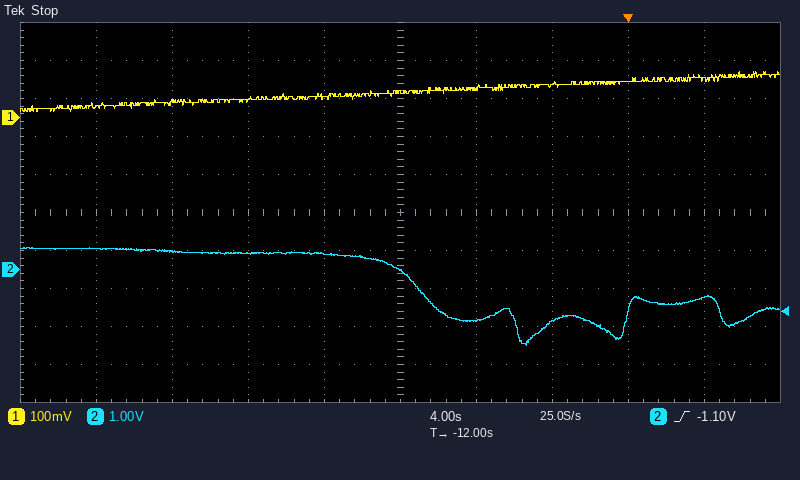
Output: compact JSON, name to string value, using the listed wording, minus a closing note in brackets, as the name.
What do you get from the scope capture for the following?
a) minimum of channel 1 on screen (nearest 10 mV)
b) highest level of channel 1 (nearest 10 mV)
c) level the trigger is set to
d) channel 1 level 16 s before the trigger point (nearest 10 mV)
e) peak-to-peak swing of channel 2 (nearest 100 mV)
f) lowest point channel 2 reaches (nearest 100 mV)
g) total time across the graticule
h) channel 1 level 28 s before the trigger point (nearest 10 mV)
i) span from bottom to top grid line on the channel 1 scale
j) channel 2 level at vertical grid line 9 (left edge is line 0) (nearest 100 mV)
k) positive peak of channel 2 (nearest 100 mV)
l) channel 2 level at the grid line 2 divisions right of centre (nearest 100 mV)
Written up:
{"minimum of channel 1 on screen": "20 mV", "highest level of channel 1": "120 mV", "level the trigger is set to": "-1.10 V", "channel 1 level 16 s before the trigger point": "60 mV", "peak-to-peak swing of channel 2": "2.6 V", "lowest point channel 2 reaches": "-2.0 V", "total time across the graticule": "40 s", "channel 1 level 28 s before the trigger point": "30 mV", "span from bottom to top grid line on the channel 1 scale": "1 V", "channel 2 level at vertical grid line 9 (left edge is line 0)": "-700 mV", "positive peak of channel 2": "600 mV", "channel 2 level at the grid line 2 divisions right of centre": "-1.4 V"}
